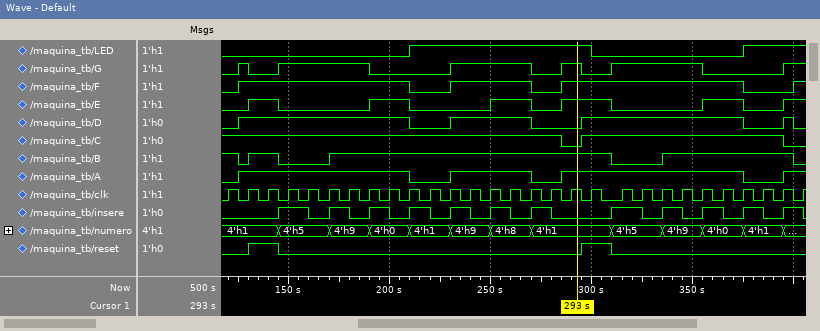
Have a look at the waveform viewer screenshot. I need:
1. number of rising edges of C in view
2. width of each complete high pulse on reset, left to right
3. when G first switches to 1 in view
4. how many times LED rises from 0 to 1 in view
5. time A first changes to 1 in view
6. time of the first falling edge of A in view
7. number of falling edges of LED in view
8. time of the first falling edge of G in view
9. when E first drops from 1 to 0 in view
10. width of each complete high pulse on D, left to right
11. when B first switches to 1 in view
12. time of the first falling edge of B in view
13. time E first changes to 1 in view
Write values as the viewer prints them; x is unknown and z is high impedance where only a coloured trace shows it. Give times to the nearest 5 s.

1
15 s, 15 s
125 s
2
125 s
210 s
1
130 s
145 s
85 s, 40 s, 80 s, 5 s
130 s
125 s
130 s
